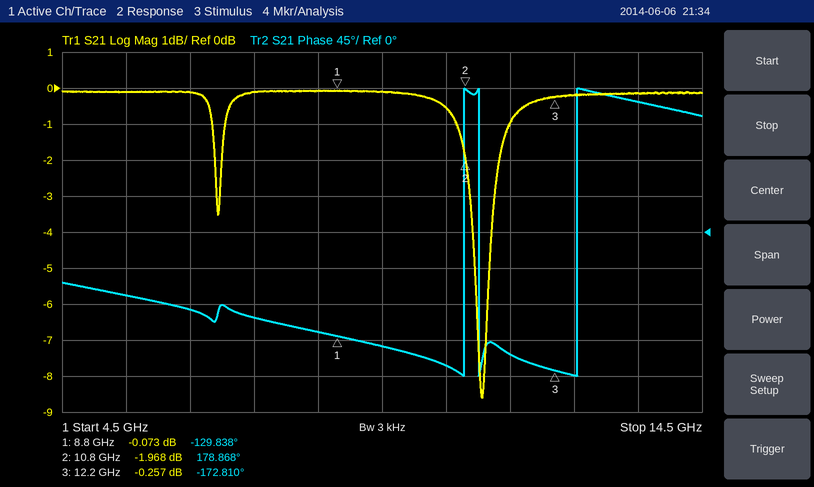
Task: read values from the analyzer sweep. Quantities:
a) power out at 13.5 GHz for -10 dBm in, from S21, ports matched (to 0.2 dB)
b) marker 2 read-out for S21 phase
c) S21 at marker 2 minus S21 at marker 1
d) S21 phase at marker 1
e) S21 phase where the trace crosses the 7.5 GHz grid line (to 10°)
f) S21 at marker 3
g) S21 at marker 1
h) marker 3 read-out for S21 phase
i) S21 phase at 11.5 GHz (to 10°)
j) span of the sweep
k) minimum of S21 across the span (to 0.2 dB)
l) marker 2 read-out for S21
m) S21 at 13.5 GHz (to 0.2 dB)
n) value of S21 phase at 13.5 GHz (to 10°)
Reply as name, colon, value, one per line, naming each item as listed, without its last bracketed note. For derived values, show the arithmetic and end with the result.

power out at 13.5 GHz for -10 dBm in, from S21, ports matched: -10 dBm + (-0.2 dB) = -10.2 dBm
marker 2 read-out for S21 phase: 178.868°
S21 at marker 2 minus S21 at marker 1: -1.968 − (-0.073) = -1.895 dB
S21 phase at marker 1: -129.838°
S21 phase where the trace crosses the 7.5 GHz grid line: -110°
S21 at marker 3: -0.257 dB
S21 at marker 1: -0.073 dB
marker 3 read-out for S21 phase: -172.810°
S21 phase at 11.5 GHz: -150°
span of the sweep: 10 GHz
minimum of S21 across the span: -8.6 dB
marker 2 read-out for S21: -1.968 dB
S21 at 13.5 GHz: -0.2 dB
value of S21 phase at 13.5 GHz: 160°
